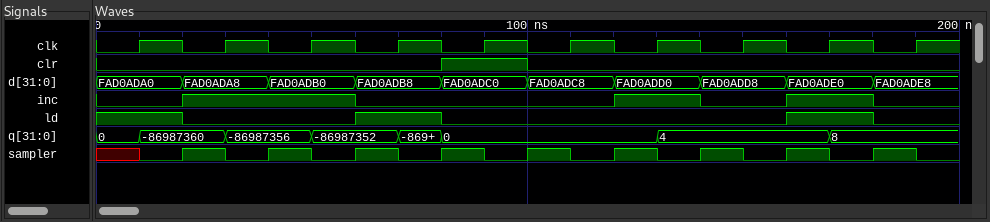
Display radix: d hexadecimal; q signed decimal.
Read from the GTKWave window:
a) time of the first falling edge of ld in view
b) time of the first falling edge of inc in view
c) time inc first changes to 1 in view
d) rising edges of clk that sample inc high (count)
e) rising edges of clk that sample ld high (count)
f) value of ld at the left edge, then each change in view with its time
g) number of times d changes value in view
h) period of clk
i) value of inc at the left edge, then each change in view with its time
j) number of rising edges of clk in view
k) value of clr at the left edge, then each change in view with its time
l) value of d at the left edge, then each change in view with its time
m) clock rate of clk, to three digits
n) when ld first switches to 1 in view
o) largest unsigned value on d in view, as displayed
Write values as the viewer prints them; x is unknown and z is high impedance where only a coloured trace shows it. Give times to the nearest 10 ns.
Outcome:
20 ns
60 ns
20 ns
4
3
1, 0 at 20 ns, 1 at 60 ns, 0 at 80 ns, 1 at 160 ns, 0 at 180 ns
9
20 ns
0, 1 at 20 ns, 0 at 60 ns, 1 at 120 ns, 0 at 140 ns, 1 at 160 ns, 0 at 180 ns
10
0, 1 at 80 ns, 0 at 100 ns
FAD0ADA0, FAD0ADA8 at 20 ns, FAD0ADB0 at 40 ns, FAD0ADB8 at 60 ns, FAD0ADC0 at 80 ns, FAD0ADC8 at 100 ns, FAD0ADD0 at 120 ns, FAD0ADD8 at 140 ns, FAD0ADE0 at 160 ns, FAD0ADE8 at 180 ns
50.0 MHz
60 ns
FAD0ADE8
